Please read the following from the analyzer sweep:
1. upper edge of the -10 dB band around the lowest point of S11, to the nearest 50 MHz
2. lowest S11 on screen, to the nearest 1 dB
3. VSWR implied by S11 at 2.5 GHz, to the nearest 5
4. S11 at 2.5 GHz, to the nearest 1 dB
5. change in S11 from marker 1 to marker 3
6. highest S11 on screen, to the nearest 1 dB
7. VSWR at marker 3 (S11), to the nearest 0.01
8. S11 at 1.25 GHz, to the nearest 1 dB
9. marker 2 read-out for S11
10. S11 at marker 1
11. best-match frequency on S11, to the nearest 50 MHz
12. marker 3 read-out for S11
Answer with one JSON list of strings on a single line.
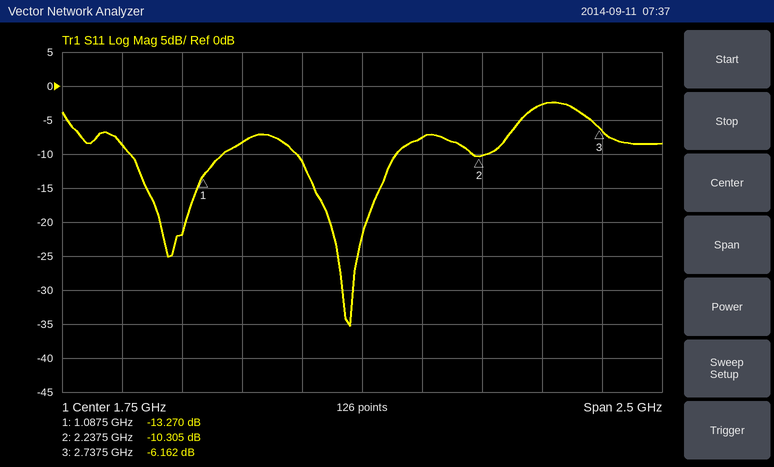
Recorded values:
["1.90 GHz", "-35 dB", "5", "-3 dB", "7.108 dB", "-2 dB", "2.94", "-8 dB", "-10.305 dB", "-13.270 dB", "1.70 GHz", "-6.162 dB"]
